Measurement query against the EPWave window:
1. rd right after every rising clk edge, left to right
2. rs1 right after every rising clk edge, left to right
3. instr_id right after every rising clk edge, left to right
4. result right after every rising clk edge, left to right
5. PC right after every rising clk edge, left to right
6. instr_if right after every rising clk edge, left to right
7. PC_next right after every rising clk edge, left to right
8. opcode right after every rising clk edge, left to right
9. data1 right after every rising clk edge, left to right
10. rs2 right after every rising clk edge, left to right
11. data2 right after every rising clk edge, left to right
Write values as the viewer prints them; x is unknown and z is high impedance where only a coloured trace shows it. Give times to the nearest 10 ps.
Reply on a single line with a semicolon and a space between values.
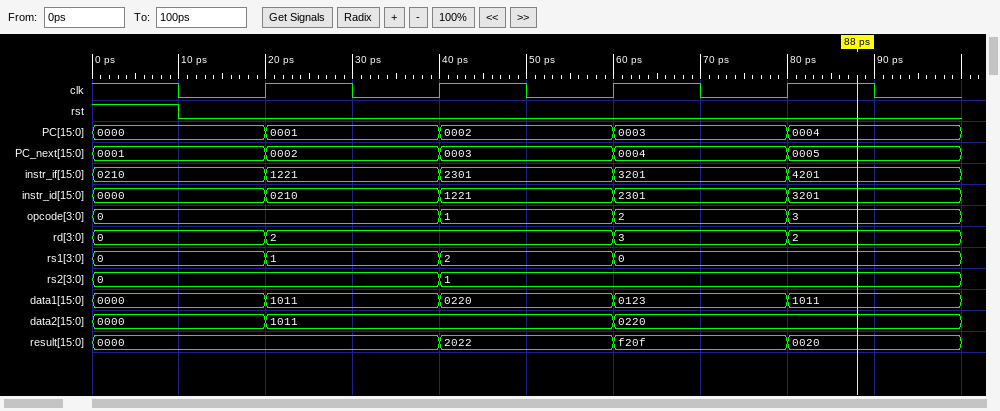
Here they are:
2, 2, 3, 2; 1, 2, 0, 0; 0210, 1221, 2301, 3201; 0000, 2022, f20f, 0020; 0001, 0002, 0003, 0004; 1221, 2301, 3201, 4201; 0002, 0003, 0004, 0005; 0, 1, 2, 3; 1011, 0220, 0123, 1011; 0, 1, 1, 1; 1011, 1011, 0220, 0220
